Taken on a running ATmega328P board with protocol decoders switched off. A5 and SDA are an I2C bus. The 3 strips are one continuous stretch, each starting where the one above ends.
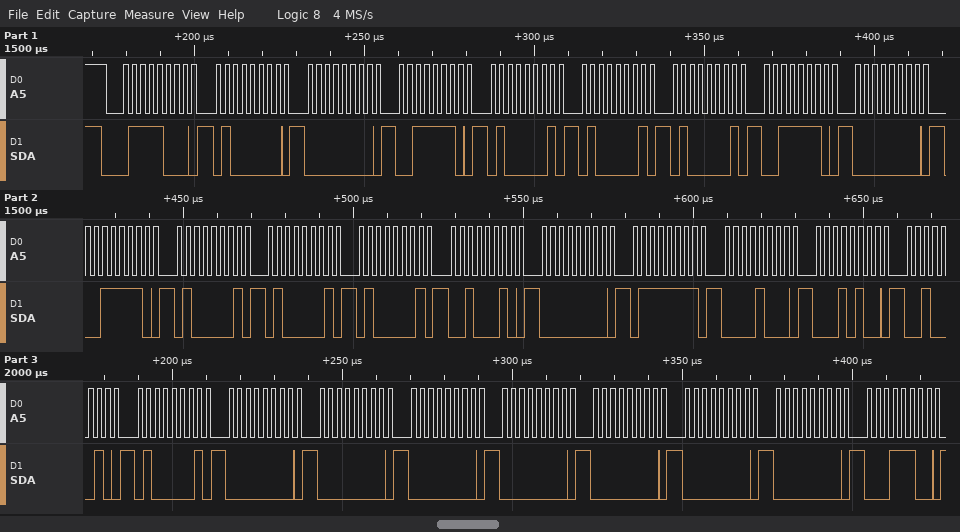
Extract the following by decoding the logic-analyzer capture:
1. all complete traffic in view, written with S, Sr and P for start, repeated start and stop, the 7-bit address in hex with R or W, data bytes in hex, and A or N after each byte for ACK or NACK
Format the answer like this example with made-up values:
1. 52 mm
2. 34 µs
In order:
1. S 3CW A 40 A 00 A 3E A 41 A 41 A 41 A 3E A 00 A 3E A 41 A 41 A 41 A 22 A 00 A 7F A 08 A 14 A 22 A 41 A 00 A 00 A 00 A 00 A 00 A 00 A 00 A 1C A
